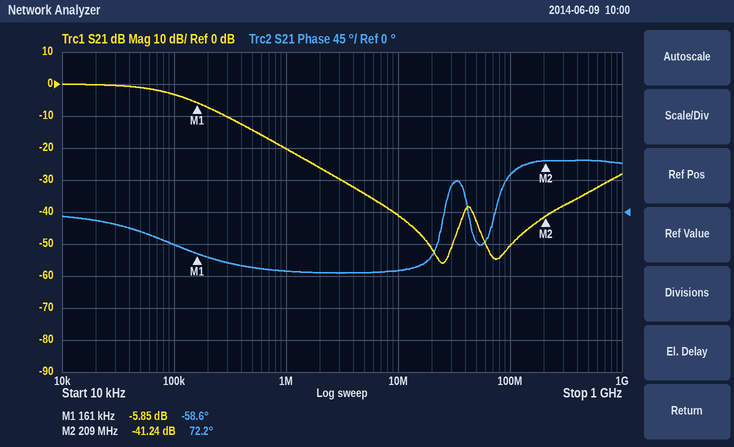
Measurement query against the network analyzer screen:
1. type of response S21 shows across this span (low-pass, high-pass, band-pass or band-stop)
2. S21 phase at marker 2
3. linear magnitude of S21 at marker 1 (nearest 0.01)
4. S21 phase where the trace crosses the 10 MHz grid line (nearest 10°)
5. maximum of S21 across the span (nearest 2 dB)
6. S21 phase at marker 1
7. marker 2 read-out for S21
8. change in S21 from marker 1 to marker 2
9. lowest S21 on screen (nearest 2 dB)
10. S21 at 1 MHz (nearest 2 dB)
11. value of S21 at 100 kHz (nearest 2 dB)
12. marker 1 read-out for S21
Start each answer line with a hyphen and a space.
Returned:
- low-pass
- 72.2°
- 0.51
- -80°
- 0 dB
- -58.6°
- -41.24 dB
- -35.39 dB
- -56 dB
- -20 dB
- -4 dB
- -5.85 dB
